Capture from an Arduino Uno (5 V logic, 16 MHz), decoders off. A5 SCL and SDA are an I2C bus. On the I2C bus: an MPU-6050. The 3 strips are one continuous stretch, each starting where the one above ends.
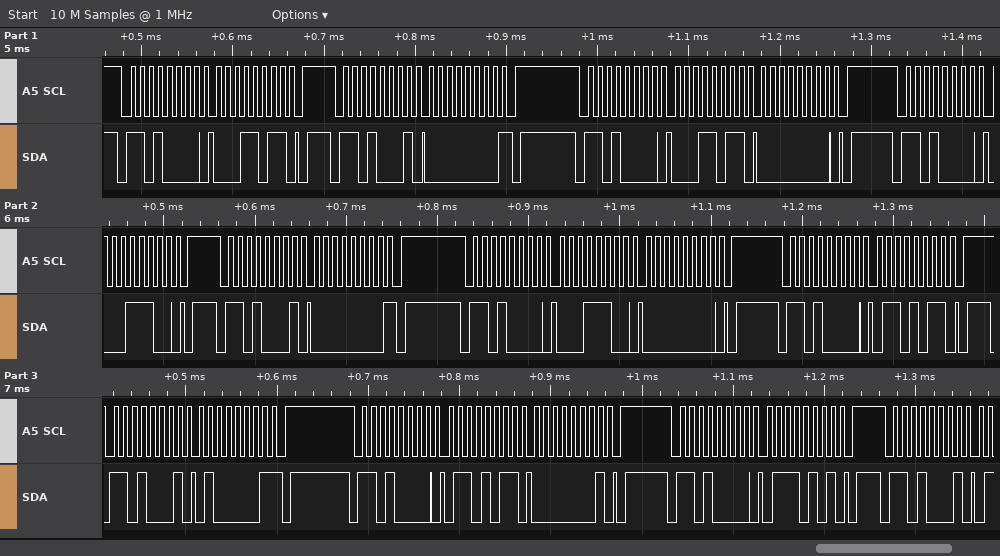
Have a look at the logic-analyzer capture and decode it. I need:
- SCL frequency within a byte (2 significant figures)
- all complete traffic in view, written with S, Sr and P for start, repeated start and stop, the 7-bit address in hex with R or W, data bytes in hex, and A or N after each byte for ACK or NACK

100 kHz
S 68W A 1B A P S 68R A 00 N P S 68W A 1B A 00 A P S 68W A 1C A P S 68R A 00 N P S 68W A 1C A 00 A P S 68W A 6B A P S 68R A 41 N P S 68W A 6B A 01 A P S 68W A 75 A P S 68R A
